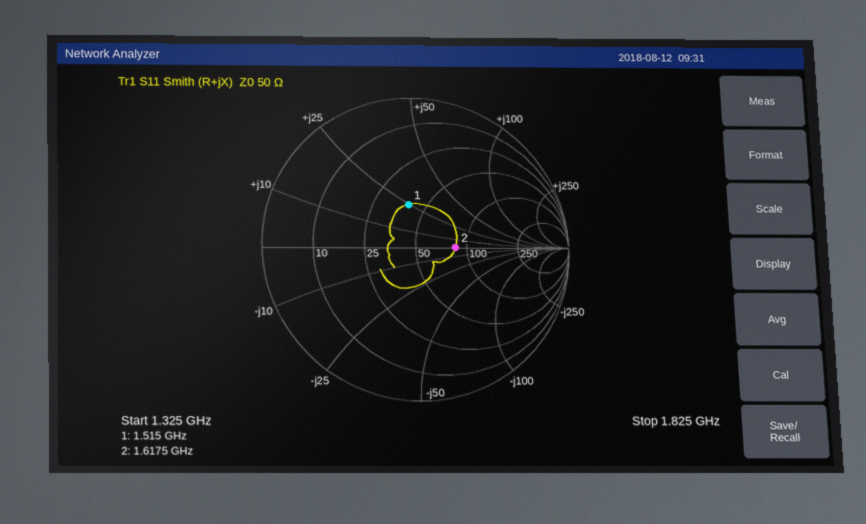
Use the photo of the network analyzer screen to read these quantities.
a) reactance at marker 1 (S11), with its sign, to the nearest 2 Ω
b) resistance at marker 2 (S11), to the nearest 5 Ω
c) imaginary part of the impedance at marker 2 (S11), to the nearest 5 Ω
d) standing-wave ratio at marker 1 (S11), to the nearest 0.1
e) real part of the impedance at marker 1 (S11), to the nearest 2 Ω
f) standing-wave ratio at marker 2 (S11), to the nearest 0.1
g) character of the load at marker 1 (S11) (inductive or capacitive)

+24 Ω
85 Ω
0 Ω
1.8
40 Ω
1.7
inductive
